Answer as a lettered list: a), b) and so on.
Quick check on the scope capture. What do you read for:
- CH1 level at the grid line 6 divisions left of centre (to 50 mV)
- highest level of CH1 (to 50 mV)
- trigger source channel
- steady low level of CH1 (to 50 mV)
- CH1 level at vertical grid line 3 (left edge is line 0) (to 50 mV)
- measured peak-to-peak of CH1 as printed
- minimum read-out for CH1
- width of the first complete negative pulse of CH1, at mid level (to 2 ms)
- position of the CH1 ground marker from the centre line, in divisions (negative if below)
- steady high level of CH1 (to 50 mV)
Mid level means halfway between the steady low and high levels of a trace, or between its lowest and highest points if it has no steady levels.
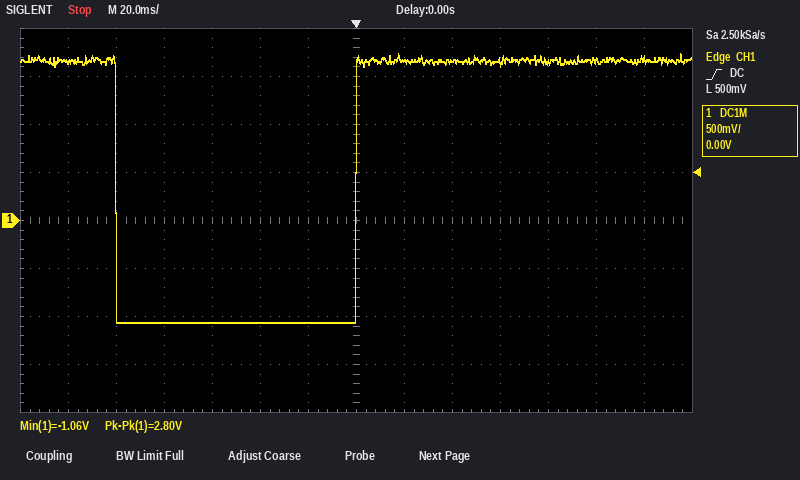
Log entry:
a) 1.65 V
b) 1.75 V
c) CH1
d) -1.05 V
e) -1.05 V
f) 2.80 V
g) -1.06 V
h) 100 ms
i) 0.0 div
j) 1.65 V
